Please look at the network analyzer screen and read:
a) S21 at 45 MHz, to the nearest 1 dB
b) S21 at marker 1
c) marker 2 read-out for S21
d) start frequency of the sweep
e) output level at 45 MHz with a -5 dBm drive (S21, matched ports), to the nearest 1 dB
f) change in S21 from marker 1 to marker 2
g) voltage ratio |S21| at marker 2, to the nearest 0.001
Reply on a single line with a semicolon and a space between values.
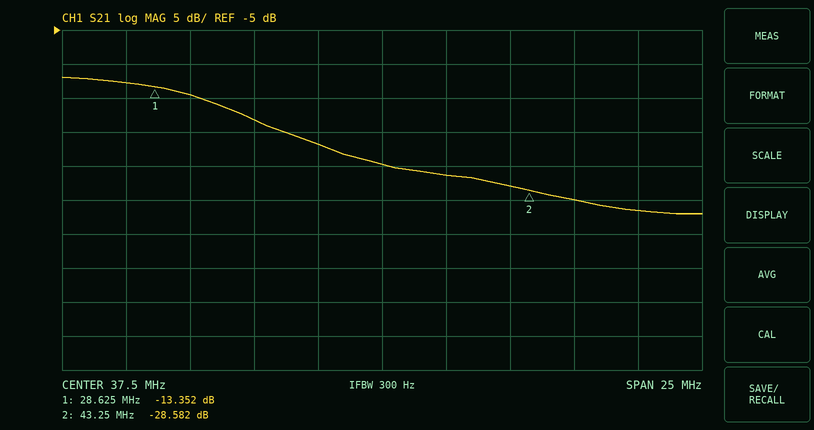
-30 dB; -13.352 dB; -28.582 dB; 25 MHz; -35 dBm; -15.230 dB; 0.037
